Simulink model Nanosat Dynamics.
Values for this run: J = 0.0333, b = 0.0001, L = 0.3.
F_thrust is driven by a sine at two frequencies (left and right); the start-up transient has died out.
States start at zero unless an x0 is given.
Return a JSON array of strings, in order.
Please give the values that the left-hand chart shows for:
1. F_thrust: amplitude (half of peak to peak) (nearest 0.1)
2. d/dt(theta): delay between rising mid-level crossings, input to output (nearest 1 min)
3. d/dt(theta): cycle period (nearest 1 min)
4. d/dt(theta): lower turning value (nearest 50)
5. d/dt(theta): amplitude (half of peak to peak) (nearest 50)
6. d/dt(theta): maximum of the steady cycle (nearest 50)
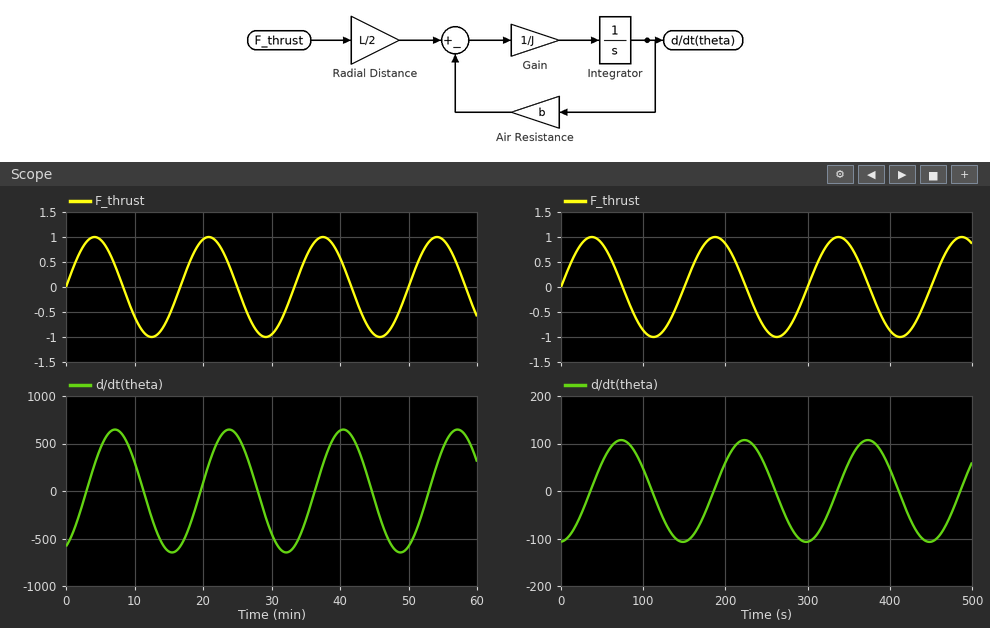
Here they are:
["1.0", "3 min", "17 min", "-650", "650", "650"]
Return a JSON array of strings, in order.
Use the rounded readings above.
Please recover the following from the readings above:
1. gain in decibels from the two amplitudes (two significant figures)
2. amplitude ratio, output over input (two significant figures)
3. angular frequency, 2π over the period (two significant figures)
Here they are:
["56 dB", "650", "0.37 rad/min"]
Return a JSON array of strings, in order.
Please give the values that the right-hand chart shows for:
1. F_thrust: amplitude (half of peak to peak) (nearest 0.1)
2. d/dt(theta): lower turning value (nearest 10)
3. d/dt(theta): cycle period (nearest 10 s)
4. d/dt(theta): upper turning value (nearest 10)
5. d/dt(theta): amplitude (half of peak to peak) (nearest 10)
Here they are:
["1.0", "-110", "150 s", "110", "110"]
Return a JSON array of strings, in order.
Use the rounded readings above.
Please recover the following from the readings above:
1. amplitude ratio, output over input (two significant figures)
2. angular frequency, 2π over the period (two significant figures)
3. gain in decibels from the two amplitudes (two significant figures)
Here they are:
["110", "0.042 rad/s", "41 dB"]
